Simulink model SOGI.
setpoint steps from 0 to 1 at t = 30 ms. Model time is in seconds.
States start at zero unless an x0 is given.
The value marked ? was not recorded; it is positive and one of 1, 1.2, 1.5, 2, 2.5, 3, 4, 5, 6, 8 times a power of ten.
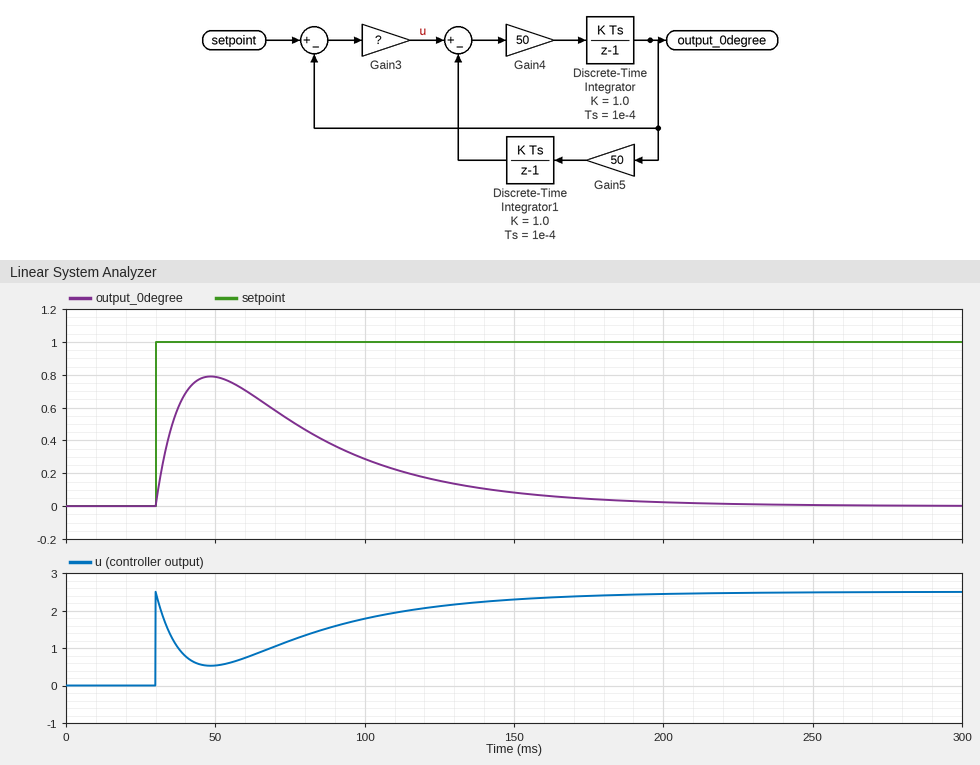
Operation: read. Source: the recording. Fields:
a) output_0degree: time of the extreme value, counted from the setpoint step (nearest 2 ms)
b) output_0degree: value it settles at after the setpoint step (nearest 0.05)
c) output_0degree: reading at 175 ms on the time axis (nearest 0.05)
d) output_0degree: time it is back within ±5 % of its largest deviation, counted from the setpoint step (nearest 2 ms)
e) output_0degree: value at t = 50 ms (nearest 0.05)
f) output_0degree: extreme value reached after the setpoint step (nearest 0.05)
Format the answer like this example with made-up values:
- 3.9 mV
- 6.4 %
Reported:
- 18 ms
- 0.00
- 0.05
- 150 ms
- 0.80
- 0.80
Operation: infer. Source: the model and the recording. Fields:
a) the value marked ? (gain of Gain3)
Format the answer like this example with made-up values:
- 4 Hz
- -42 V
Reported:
- 2.5
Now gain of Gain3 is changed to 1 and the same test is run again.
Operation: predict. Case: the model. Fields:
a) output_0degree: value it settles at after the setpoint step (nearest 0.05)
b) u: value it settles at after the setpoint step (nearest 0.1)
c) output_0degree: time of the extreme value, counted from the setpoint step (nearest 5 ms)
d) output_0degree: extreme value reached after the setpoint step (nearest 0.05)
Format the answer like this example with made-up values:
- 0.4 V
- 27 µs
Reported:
- 0.00
- 1.0
- 25 ms
- 0.55
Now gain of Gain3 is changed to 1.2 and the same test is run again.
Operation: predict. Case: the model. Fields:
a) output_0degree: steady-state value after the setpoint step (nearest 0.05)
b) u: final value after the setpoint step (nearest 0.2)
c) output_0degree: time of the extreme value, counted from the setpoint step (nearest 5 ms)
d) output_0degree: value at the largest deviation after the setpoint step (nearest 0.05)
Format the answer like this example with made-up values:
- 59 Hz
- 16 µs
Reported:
- 0.00
- 1.2
- 25 ms
- 0.60
